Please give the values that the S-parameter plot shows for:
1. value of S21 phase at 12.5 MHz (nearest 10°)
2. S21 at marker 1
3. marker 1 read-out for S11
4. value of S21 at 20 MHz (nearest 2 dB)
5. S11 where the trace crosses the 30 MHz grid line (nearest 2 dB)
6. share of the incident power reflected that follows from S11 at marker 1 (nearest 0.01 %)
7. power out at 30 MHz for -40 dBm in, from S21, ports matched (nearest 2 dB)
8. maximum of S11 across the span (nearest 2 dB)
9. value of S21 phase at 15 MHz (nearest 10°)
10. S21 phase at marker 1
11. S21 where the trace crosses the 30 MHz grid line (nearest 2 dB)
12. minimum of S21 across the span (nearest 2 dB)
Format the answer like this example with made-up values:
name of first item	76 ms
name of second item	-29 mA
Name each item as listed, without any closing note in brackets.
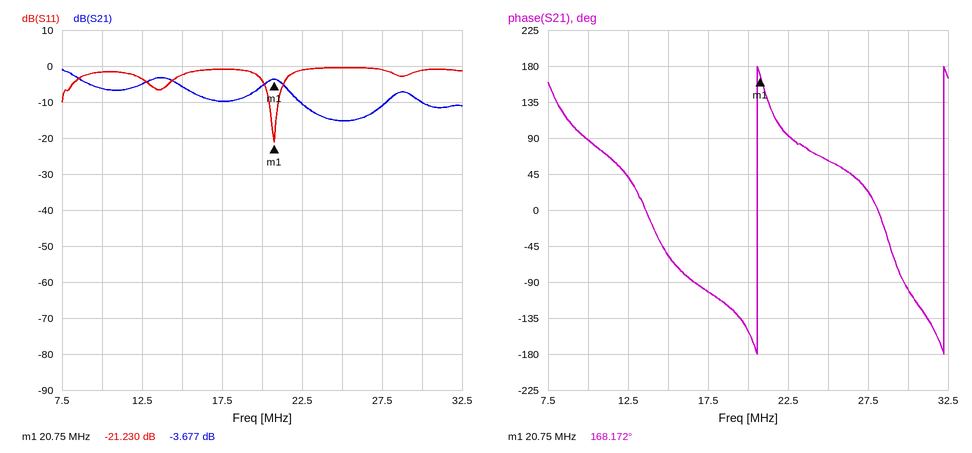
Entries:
value of S21 phase at 12.5 MHz	40°
S21 at marker 1	-3.677 dB
marker 1 read-out for S11	-21.230 dB
value of S21 at 20 MHz	-6 dB
S11 where the trace crosses the 30 MHz grid line	-2 dB
share of the incident power reflected that follows from S11 at marker 1	0.75 %
power out at 30 MHz for -40 dBm in, from S21, ports matched	-50 dBm
maximum of S11 across the span	0 dB
value of S21 phase at 15 MHz	-60°
S21 phase at marker 1	168.172°
S21 where the trace crosses the 30 MHz grid line	-10 dB
minimum of S21 across the span	-16 dB
